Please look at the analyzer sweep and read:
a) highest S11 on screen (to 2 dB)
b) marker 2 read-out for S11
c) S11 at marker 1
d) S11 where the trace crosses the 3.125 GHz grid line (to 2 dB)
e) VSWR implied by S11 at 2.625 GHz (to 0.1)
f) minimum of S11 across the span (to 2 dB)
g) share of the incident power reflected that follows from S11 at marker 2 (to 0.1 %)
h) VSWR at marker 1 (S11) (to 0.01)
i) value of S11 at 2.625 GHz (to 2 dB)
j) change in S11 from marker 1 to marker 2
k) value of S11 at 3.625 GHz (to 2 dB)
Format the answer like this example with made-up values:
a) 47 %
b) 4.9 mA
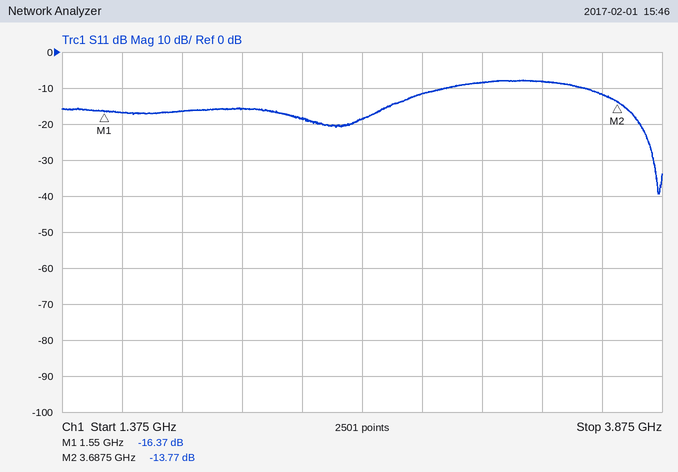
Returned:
a) -8 dB
b) -13.77 dB
c) -16.37 dB
d) -8 dB
e) 1.3
f) -40 dB
g) 4.2 %
h) 1.36
i) -18 dB
j) 2.60 dB
k) -12 dB
